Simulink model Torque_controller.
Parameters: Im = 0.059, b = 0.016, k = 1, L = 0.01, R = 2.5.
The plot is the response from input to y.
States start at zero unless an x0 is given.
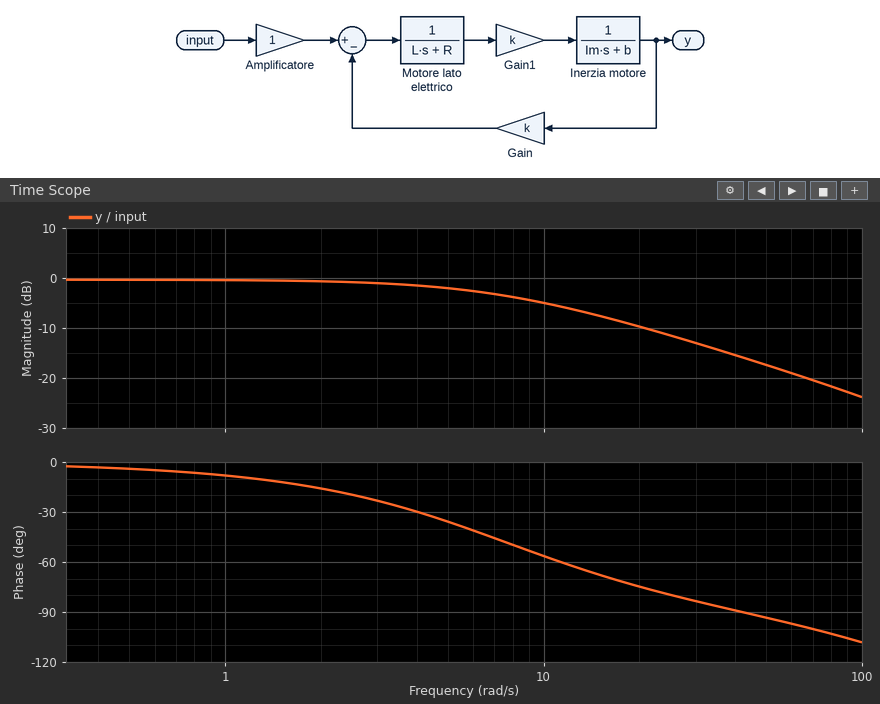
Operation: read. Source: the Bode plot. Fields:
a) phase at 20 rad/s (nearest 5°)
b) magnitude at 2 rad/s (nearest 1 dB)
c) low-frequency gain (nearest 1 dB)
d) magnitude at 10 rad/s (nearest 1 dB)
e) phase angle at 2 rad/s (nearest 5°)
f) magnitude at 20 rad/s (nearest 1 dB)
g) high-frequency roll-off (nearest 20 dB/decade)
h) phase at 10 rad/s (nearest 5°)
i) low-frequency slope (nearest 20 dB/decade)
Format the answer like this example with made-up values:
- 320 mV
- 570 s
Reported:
- -75°
- -1 dB
- 0 dB
- -5 dB
- -15°
- -10 dB
- -20 dB/decade
- -55°
- 0 dB/decade
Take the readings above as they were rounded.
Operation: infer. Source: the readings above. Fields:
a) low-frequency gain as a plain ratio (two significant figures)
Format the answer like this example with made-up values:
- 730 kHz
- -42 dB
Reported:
- 1.0
